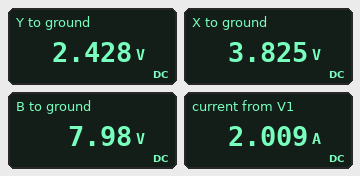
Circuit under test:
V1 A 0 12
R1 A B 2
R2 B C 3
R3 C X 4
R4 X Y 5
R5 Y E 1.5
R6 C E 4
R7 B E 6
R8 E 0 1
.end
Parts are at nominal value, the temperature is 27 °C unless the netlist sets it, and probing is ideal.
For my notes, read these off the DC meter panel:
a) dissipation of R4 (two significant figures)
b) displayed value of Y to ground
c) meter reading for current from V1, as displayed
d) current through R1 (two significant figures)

390 mW
2.428 V
2.009 A
2.0 A
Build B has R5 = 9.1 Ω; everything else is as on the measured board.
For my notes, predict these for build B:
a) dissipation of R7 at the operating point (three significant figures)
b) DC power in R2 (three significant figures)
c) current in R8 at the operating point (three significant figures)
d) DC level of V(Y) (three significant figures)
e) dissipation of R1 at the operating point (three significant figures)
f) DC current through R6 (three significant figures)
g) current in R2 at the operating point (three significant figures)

6.13 W
2.80 W
1.98 A
3.57 V
7.82 W
792 mA
967 mA
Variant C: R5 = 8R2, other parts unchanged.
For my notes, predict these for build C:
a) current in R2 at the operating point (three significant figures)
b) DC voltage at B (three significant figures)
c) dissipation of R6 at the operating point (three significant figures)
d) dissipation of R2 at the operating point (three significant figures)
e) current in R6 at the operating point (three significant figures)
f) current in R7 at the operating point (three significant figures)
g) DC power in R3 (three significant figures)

970 mA
8.04 V
2.48 W
2.82 W
787 mA
1.01 A
134 mW
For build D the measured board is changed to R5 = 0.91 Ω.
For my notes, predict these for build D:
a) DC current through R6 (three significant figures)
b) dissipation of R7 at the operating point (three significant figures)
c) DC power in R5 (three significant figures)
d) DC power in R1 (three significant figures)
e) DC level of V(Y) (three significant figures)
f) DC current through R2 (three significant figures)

726 mA
5.92 W
78.2 mW
8.10 W
2.28 V
1.02 A
